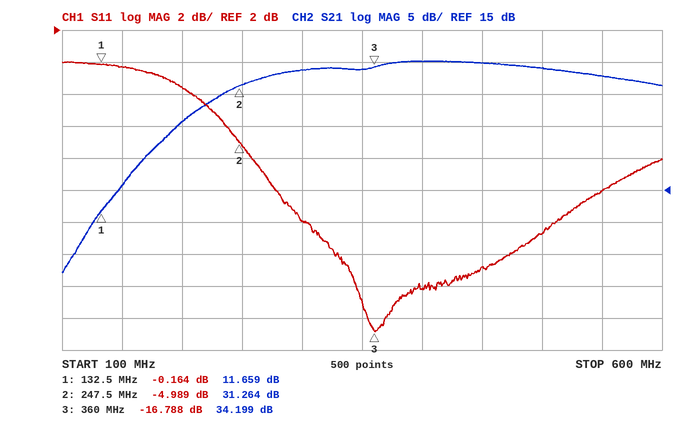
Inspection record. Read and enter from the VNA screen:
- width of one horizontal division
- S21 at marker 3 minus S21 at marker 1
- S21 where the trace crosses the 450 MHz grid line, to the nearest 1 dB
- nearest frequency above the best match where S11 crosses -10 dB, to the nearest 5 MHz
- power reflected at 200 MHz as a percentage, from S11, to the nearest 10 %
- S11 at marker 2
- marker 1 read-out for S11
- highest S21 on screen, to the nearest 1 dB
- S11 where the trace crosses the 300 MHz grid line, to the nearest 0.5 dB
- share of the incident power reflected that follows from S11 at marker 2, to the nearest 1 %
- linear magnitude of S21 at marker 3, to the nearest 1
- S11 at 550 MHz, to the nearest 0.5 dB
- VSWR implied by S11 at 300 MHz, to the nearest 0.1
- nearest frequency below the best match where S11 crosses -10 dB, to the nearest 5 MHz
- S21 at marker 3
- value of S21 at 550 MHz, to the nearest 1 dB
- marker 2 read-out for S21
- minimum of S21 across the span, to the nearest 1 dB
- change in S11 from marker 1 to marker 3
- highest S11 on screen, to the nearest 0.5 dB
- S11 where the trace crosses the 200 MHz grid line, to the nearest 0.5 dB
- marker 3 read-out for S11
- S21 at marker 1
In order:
50 MHz
22.540 dB
35 dB
510 MHz
70 %
-4.989 dB
-0.164 dB
35 dB
-10.0 dB
32 %
51
-8.0 dB
1.9
305 MHz
34.199 dB
33 dB
31.264 dB
2 dB
-16.624 dB
0.0 dB
-1.5 dB
-16.788 dB
11.659 dB
